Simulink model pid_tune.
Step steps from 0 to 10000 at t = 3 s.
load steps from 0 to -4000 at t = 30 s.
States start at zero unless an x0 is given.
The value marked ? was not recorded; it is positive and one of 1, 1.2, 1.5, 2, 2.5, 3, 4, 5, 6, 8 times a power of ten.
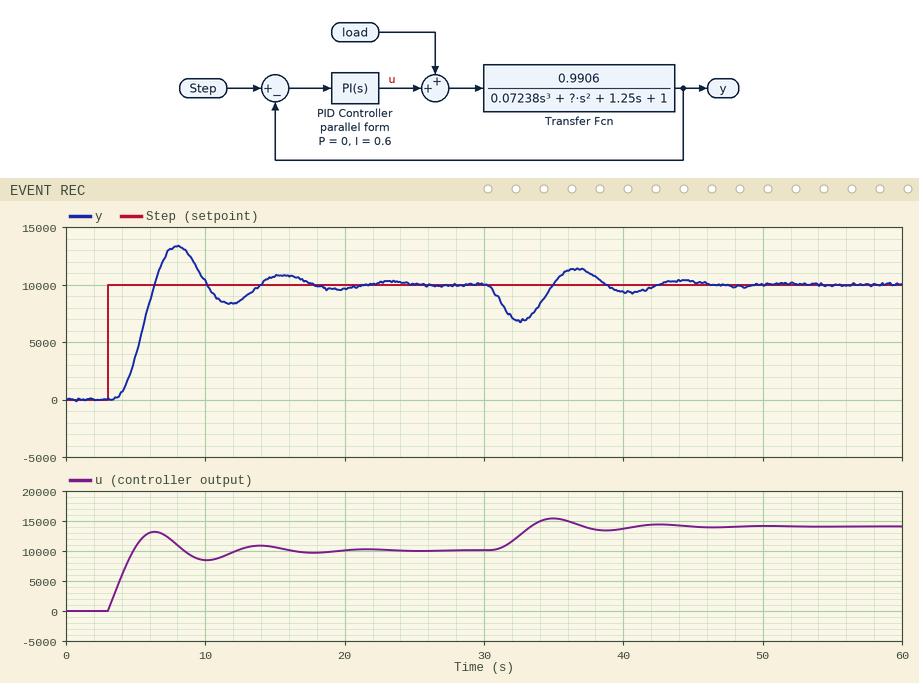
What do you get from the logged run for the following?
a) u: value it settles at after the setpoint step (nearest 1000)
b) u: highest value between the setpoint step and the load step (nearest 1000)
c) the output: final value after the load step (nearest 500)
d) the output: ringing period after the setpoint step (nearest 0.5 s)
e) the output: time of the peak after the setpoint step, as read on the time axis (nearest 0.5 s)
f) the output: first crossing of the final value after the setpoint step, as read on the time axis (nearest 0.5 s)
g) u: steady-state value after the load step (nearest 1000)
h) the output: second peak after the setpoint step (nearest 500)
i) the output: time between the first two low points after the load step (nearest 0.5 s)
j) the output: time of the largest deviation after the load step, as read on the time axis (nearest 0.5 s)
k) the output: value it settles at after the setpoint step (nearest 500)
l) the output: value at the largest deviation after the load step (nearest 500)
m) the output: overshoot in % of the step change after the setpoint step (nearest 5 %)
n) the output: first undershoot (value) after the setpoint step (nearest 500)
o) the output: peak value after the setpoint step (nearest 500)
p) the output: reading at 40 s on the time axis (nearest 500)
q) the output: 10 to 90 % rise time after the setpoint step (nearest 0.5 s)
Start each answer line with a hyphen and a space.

- 10000
- 13000
- 10000
- 7.5 s
- 8.0 s
- 6.5 s
- 14000
- 11000
- 8.0 s
- 32.5 s
- 10000
- 7000
- 35 %
- 8500
- 13500
- 9500
- 2.0 s
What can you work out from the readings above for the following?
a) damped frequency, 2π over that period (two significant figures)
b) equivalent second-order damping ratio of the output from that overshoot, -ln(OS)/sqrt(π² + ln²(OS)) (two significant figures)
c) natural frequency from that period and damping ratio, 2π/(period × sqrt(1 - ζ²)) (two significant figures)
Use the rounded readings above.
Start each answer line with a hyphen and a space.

- 0.84 rad/s
- 0.32
- 0.88 rad/s
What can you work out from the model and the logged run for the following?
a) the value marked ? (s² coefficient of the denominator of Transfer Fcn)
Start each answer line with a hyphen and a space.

- 1
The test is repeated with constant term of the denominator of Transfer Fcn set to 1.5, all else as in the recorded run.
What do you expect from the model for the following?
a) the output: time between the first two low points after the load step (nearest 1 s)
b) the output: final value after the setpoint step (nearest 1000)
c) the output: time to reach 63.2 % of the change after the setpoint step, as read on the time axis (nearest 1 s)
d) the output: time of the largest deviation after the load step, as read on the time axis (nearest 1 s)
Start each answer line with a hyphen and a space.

- 6 s
- 10000
- 6 s
- 32 s
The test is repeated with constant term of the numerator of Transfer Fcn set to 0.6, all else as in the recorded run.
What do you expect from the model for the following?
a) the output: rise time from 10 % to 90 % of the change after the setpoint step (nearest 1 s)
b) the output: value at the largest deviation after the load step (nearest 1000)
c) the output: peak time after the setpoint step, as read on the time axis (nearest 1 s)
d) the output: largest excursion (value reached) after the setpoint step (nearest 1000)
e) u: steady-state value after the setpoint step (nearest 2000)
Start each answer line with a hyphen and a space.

- 3 s
- 8000
- 9 s
- 11000
- 16000
